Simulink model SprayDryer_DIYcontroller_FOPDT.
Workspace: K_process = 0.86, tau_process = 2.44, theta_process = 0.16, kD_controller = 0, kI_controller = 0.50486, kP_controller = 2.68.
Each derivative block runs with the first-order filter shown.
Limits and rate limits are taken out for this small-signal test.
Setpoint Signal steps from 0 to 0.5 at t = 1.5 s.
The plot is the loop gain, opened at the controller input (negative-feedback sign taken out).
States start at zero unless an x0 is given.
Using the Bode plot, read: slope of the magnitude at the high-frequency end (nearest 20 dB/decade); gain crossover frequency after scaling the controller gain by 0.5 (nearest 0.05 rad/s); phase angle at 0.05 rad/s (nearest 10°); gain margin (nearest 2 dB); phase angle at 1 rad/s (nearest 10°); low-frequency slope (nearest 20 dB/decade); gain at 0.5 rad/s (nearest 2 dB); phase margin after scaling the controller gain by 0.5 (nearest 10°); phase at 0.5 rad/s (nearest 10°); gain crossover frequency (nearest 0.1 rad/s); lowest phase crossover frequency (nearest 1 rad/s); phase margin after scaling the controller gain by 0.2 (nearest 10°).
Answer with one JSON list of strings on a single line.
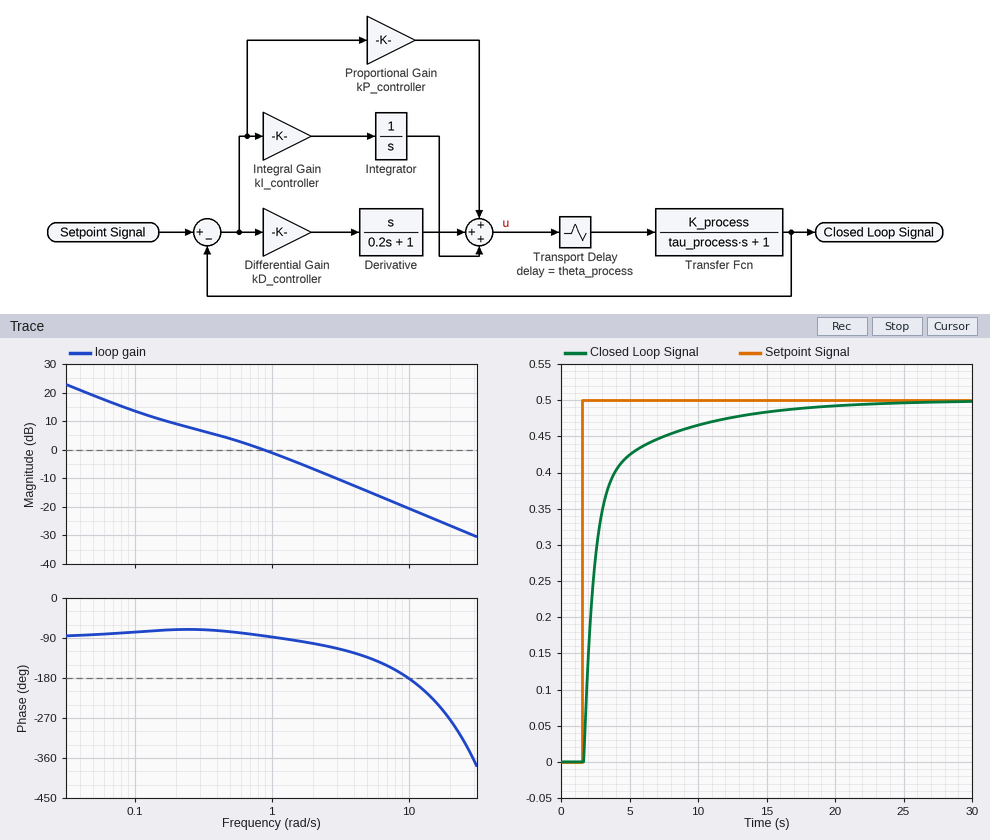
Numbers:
["-20 dB/decade", "0.35 rad/s", "-80°", "20 dB", "-90°", "-20 dB/decade", "4 dB", "110°", "-80°", "0.9 rad/s", "10 rad/s", "100°"]
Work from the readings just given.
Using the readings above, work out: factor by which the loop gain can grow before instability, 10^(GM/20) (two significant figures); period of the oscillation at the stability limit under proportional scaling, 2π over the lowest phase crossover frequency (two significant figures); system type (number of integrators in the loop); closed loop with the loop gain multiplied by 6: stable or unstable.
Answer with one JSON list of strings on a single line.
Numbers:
["10", "0.63 s", "1", "stable"]
